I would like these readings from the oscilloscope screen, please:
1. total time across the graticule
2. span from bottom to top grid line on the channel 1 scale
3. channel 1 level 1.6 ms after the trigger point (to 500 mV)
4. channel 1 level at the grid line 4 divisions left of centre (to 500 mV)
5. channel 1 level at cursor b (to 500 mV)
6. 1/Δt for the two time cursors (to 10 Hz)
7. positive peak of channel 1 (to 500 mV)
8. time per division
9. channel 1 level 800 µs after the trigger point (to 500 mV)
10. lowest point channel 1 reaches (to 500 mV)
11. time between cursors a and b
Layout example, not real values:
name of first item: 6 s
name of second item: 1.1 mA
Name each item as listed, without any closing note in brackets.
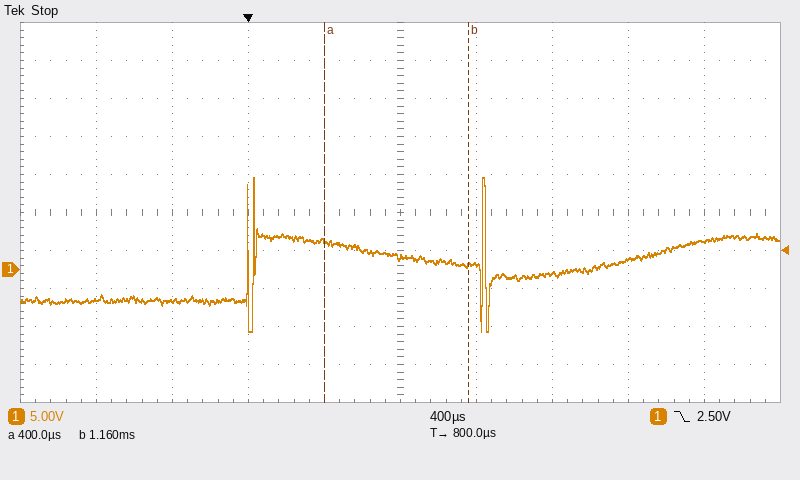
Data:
total time across the graticule: 4 ms
span from bottom to top grid line on the channel 1 scale: 50 V
channel 1 level 1.6 ms after the trigger point: -500 mV
channel 1 level at the grid line 4 divisions left of centre: -4.0 V
channel 1 level at cursor b: 500 mV
1/Δt for the two time cursors: 1.32 kHz
positive peak of channel 1: 12.0 V
time per division: 400 µs
channel 1 level 800 µs after the trigger point: 1.5 V
lowest point channel 1 reaches: -8.0 V
time between cursors a and b: 760 µs
